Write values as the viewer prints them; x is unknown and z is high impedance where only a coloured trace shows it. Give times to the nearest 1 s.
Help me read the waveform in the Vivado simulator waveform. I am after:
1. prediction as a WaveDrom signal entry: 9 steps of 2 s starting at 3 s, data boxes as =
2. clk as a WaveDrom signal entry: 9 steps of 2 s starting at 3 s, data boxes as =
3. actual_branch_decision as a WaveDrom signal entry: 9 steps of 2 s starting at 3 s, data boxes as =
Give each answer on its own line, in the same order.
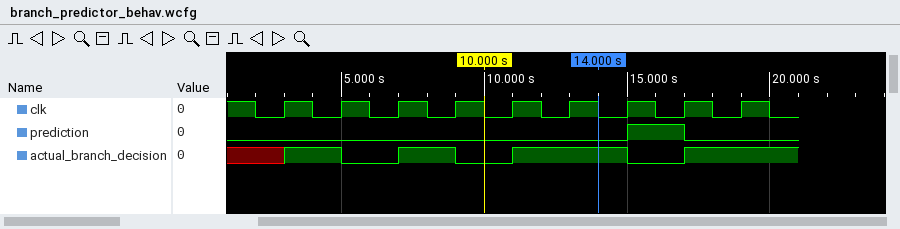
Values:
{name: 'prediction', wave: '0.....10.'}
{name: 'clk', wave: 'p........'}
{name: 'actual_branch_decision', wave: '10101.01.'}
